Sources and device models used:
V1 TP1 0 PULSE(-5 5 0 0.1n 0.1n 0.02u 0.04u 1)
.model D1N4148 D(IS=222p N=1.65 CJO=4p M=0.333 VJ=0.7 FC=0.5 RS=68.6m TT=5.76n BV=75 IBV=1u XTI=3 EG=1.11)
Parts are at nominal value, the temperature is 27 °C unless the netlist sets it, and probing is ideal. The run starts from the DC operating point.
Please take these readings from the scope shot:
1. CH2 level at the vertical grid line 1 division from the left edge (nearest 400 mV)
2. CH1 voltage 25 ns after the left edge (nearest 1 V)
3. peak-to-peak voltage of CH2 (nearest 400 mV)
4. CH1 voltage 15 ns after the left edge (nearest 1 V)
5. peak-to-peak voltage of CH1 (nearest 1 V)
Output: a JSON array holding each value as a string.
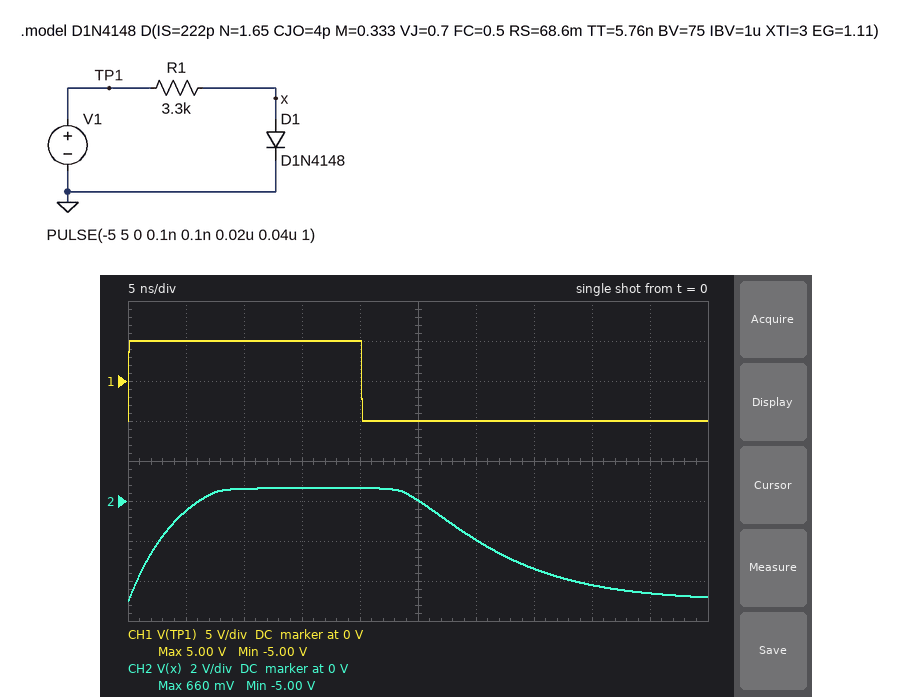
["-400 mV", "-5 V", "5.6 V", "5 V", "10 V"]
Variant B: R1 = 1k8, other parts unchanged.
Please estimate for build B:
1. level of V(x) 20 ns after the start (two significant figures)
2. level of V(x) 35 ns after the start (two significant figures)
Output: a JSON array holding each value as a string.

["690 mV", "-4.6 V"]
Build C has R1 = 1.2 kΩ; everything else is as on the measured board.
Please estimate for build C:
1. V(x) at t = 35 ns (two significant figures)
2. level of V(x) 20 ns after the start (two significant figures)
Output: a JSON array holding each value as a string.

["-4.9 V", "710 mV"]
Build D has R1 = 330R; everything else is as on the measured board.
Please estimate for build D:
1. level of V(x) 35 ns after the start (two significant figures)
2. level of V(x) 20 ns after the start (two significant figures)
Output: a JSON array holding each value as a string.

["-5.0 V", "760 mV"]
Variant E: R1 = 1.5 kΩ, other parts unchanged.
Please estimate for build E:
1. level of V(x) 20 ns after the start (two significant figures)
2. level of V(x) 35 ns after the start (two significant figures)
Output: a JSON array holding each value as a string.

["700 mV", "-4.8 V"]
